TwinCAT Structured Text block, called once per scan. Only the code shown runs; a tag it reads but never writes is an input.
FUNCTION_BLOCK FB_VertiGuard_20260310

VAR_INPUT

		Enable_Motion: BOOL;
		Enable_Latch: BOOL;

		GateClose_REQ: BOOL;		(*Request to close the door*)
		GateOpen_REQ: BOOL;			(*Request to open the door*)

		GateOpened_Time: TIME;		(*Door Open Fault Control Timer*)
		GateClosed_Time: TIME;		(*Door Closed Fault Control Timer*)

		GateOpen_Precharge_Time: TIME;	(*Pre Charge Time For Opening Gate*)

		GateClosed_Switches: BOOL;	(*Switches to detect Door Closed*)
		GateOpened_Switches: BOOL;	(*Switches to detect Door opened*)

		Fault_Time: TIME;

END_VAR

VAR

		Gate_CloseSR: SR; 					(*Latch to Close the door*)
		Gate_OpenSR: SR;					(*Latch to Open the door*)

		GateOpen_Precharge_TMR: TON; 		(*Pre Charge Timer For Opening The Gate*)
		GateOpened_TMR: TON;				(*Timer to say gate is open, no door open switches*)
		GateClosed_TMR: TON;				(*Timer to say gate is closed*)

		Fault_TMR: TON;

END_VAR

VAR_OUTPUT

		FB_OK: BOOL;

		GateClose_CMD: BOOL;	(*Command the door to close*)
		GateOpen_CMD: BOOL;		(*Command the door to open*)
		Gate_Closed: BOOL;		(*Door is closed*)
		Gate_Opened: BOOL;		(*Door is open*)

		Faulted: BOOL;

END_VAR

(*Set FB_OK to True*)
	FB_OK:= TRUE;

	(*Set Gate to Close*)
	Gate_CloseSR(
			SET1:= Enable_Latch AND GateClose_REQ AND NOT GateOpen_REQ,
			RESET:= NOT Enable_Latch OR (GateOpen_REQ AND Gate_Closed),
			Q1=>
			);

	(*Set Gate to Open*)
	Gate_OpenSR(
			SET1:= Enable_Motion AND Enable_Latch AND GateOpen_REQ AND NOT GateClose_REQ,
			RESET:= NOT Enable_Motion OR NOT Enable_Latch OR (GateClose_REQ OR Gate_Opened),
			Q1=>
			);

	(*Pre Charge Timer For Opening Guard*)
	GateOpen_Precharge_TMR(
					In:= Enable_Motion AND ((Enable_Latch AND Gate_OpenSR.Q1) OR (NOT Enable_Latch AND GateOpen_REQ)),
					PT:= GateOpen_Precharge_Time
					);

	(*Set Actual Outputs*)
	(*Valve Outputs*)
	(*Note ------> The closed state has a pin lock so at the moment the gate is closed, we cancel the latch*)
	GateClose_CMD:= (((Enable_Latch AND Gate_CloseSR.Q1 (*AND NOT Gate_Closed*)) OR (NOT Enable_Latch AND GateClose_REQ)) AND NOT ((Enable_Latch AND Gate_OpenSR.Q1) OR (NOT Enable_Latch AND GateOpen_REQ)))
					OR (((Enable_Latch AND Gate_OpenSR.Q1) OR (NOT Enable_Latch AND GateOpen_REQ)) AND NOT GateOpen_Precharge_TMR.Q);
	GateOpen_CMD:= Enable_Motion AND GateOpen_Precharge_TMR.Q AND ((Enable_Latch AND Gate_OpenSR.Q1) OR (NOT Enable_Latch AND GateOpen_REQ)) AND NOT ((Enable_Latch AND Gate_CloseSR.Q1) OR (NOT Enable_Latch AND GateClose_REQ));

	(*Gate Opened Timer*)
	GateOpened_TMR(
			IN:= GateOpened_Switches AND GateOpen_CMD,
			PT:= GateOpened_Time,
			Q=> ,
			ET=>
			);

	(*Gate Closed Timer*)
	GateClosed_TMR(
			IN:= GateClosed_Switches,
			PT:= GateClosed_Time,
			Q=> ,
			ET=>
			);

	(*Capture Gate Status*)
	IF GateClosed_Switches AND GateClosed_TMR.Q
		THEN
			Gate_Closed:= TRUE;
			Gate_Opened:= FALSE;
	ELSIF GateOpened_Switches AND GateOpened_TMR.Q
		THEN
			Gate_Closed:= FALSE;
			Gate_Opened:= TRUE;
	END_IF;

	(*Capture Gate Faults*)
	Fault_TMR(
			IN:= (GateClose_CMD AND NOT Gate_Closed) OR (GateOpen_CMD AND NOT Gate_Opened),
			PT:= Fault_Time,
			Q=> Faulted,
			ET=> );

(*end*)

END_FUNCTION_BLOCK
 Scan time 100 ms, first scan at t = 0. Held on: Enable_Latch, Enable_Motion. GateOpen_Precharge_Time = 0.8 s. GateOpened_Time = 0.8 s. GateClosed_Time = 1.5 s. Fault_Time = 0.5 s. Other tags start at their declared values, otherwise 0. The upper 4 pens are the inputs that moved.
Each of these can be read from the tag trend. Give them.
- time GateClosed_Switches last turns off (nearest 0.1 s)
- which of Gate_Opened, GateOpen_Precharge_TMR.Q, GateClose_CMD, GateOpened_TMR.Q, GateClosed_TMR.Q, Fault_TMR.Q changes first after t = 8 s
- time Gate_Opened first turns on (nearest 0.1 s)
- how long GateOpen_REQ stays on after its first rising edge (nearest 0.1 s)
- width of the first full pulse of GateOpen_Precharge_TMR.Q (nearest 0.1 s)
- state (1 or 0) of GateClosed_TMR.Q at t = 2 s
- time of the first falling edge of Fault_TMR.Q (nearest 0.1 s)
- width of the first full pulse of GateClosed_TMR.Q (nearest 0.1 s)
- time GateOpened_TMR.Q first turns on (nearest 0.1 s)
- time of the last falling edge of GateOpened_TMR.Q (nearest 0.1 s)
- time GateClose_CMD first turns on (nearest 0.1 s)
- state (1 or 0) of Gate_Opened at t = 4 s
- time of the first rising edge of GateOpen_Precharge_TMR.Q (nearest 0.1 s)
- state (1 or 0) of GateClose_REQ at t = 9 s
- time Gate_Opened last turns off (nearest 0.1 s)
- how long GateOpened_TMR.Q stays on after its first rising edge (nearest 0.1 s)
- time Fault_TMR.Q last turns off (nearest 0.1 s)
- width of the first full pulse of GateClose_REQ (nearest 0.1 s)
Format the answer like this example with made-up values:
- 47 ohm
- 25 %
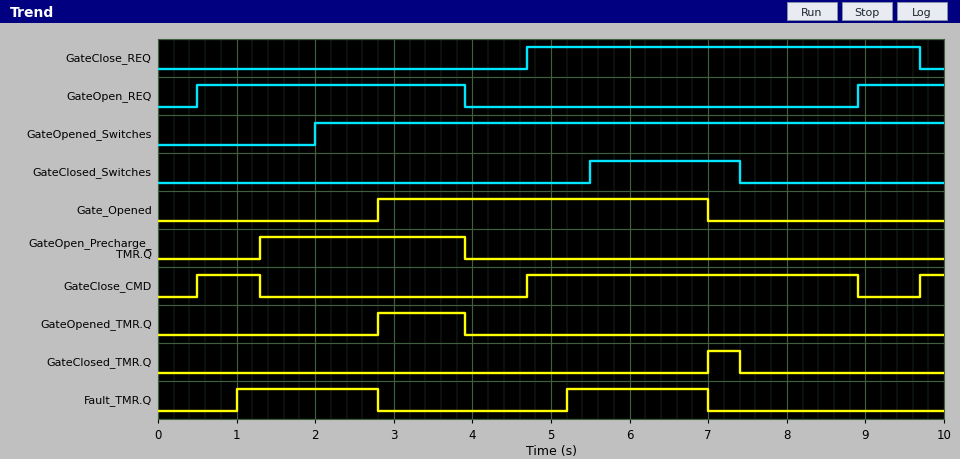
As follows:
- 7.4 s
- GateClose_CMD
- 2.8 s
- 3.4 s
- 2.6 s
- 0
- 2.8 s
- 0.4 s
- 2.8 s
- 3.9 s
- 0.5 s
- 1
- 1.3 s
- 1
- 7.0 s
- 1.1 s
- 7.0 s
- 5.0 s
